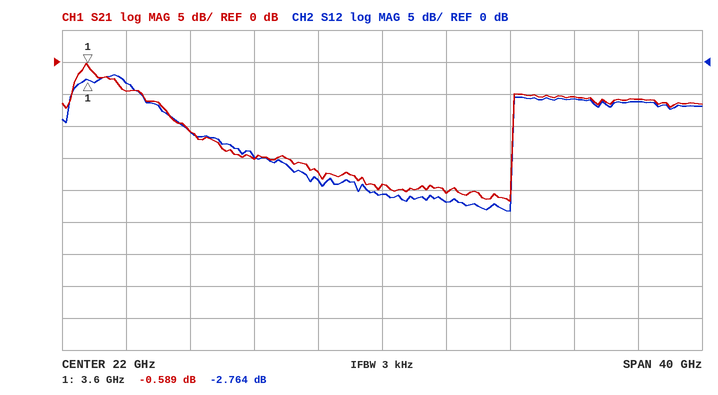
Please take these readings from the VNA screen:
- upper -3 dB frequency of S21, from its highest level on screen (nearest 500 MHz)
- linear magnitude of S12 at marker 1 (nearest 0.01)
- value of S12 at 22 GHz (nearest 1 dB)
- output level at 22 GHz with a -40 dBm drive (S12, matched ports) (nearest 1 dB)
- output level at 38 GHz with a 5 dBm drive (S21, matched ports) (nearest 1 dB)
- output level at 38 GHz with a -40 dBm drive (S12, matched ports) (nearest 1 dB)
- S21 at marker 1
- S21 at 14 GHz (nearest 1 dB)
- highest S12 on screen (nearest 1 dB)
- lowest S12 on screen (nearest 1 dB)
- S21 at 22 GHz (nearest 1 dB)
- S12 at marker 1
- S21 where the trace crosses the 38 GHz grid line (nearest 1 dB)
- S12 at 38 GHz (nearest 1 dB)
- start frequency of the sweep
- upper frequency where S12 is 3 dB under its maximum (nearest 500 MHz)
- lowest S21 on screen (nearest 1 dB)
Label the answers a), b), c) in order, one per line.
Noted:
a) 5.5 GHz
b) 0.73
c) -21 dB
d) -61 dBm
e) -1 dBm
f) -46 dBm
g) -0.589 dB
h) -15 dB
i) -2 dB
j) -23 dB
k) -19 dB
l) -2.764 dB
m) -6 dB
n) -6 dB
o) 2 GHz
p) 7.0 GHz
q) -22 dB
